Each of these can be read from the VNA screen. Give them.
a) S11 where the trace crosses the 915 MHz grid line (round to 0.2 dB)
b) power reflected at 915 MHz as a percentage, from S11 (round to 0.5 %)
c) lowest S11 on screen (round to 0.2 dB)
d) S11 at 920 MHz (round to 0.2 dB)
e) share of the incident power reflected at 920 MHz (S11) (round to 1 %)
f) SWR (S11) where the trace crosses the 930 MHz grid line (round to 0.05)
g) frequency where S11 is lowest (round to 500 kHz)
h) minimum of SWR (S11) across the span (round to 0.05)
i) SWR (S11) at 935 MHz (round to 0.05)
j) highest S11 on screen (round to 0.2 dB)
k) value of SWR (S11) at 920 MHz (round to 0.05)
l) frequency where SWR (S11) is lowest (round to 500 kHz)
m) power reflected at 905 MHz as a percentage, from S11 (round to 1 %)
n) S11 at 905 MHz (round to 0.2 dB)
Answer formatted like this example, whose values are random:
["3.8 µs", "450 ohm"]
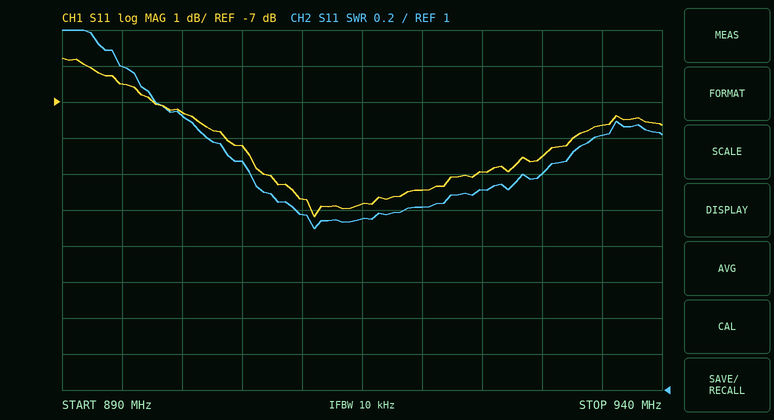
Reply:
["-9.8 dB", "10.5 %", "-10.2 dB", "-9.4 dB", "11 %", "2.20", "911.0 MHz", "1.90", "2.40", "-5.8 dB", "2.00", "911.0 MHz", "15 %", "-8.2 dB"]
